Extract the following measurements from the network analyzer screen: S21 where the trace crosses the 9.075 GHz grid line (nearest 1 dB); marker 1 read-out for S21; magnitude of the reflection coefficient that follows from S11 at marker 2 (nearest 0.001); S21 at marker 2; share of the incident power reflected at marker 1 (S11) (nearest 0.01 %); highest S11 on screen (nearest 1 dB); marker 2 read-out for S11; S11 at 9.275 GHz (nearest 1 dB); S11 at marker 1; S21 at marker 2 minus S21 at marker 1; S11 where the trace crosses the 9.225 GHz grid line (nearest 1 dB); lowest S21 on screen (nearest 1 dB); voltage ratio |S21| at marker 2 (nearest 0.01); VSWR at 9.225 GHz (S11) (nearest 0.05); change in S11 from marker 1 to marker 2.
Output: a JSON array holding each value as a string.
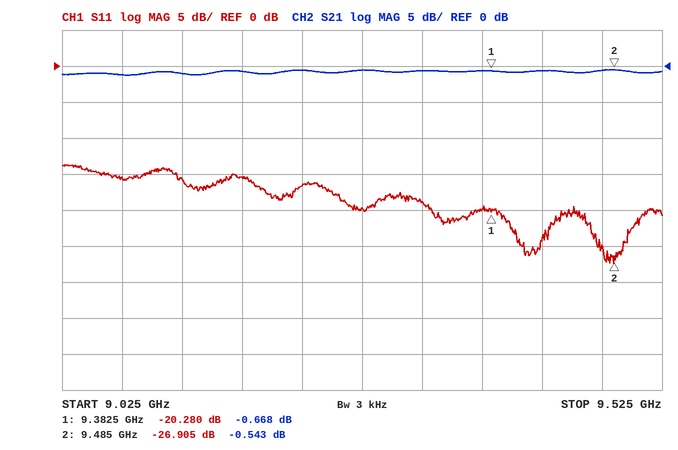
["-1 dB", "-0.668 dB", "0.045", "-0.543 dB", "0.94 %", "-14 dB", "-26.905 dB", "-20 dB", "-20.280 dB", "0.125 dB", "-17 dB", "-1 dB", "0.94", "1.35", "-6.625 dB"]
